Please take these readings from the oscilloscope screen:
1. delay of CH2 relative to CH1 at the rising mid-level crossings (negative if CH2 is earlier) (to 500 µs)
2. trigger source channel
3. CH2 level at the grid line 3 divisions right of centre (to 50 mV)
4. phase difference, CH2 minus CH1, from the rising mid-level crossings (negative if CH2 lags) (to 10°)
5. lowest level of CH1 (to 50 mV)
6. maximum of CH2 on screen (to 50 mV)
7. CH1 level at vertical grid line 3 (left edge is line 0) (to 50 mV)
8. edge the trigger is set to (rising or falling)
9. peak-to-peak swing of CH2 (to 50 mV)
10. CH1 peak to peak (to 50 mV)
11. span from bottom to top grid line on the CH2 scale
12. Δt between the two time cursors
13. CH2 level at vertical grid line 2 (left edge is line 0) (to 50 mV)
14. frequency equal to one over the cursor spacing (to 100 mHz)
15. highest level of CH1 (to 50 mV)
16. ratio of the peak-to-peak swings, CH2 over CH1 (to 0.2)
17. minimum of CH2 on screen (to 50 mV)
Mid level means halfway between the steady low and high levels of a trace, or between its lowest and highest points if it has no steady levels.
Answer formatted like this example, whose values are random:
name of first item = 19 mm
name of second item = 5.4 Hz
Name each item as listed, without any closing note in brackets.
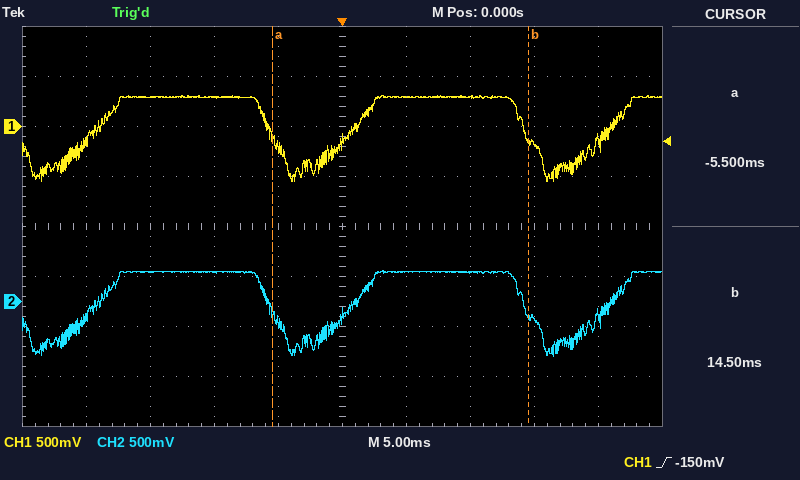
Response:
delay of CH2 relative to CH1 at the rising mid-level crossings (negative if CH2 is earlier) = 0.0 ms
trigger source channel = CH1
CH2 level at the grid line 3 divisions right of centre = -150 mV
phase difference, CH2 minus CH1, from the rising mid-level crossings (negative if CH2 lags) = 0°
lowest level of CH1 = -550 mV
maximum of CH2 on screen = 300 mV
CH1 level at vertical grid line 3 (left edge is line 0) = 300 mV
edge the trigger is set to = rising
peak-to-peak swing of CH2 = 850 mV
CH1 peak to peak = 850 mV
span from bottom to top grid line on the CH2 scale = 4 V
Δt between the two time cursors = 20.0 ms
CH2 level at vertical grid line 2 (left edge is line 0) = 300 mV
frequency equal to one over the cursor spacing = 50.0 Hz
highest level of CH1 = 300 mV
ratio of the peak-to-peak swings, CH2 over CH1 = 1.0
minimum of CH2 on screen = -550 mV
